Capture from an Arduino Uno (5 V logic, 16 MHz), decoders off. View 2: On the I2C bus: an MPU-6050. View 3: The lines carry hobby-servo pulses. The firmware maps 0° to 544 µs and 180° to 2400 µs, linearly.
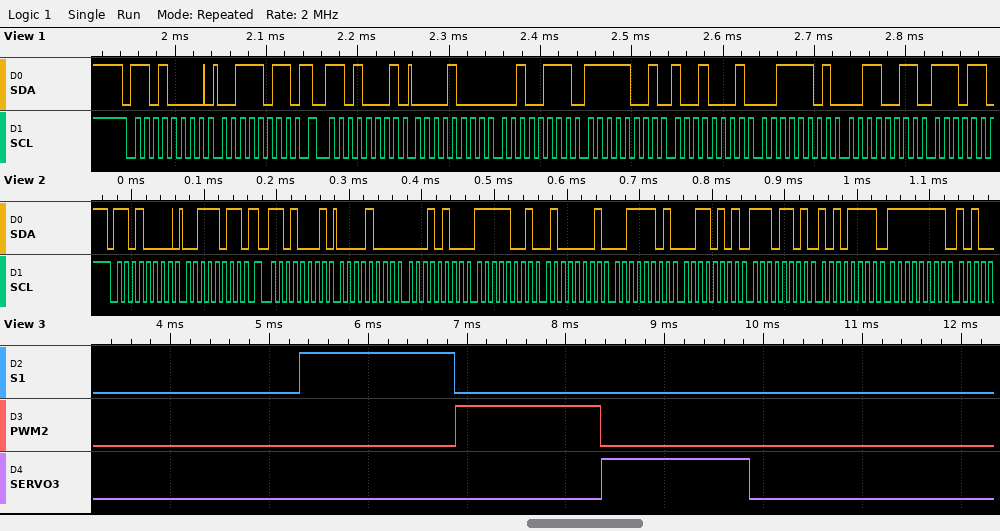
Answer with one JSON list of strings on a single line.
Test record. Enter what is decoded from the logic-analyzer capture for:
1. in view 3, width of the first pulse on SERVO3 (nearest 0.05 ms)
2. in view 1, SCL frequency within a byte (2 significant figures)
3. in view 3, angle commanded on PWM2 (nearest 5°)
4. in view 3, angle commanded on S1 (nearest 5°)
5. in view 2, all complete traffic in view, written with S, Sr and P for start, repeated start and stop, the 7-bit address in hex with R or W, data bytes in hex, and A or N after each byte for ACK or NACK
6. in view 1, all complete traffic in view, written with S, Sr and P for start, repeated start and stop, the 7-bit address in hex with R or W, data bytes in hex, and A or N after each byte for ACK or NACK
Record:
["1.50 ms", "100 kHz", "90°", "100°", "S 68W A 3B A Sr 68R A 08 A 14 A F9 A 41 A 3D A 35 A ED A AF A FF A", "S 68W A 3B A Sr 68R A 08 A 27 A F9 A 91 A 3D A 33 A"]
